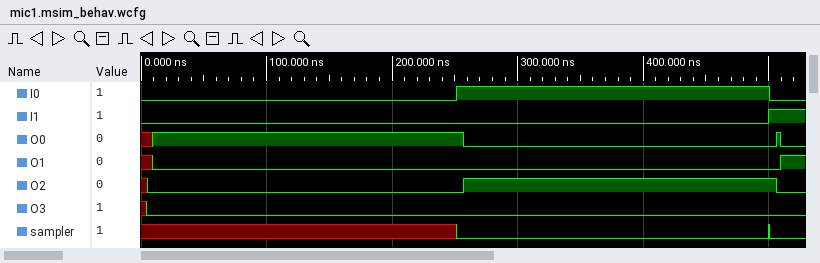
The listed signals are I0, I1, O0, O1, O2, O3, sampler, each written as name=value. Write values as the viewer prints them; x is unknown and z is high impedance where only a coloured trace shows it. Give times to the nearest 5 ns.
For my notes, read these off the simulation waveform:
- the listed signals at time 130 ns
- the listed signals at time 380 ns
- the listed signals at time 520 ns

I0=0, I1=0, O0=1, O1=0, O2=0, O3=0, sampler=x
I0=1, I1=0, O0=0, O1=0, O2=1, O3=0, sampler=0
I0=0, I1=1, O0=0, O1=1, O2=0, O3=0, sampler=0
